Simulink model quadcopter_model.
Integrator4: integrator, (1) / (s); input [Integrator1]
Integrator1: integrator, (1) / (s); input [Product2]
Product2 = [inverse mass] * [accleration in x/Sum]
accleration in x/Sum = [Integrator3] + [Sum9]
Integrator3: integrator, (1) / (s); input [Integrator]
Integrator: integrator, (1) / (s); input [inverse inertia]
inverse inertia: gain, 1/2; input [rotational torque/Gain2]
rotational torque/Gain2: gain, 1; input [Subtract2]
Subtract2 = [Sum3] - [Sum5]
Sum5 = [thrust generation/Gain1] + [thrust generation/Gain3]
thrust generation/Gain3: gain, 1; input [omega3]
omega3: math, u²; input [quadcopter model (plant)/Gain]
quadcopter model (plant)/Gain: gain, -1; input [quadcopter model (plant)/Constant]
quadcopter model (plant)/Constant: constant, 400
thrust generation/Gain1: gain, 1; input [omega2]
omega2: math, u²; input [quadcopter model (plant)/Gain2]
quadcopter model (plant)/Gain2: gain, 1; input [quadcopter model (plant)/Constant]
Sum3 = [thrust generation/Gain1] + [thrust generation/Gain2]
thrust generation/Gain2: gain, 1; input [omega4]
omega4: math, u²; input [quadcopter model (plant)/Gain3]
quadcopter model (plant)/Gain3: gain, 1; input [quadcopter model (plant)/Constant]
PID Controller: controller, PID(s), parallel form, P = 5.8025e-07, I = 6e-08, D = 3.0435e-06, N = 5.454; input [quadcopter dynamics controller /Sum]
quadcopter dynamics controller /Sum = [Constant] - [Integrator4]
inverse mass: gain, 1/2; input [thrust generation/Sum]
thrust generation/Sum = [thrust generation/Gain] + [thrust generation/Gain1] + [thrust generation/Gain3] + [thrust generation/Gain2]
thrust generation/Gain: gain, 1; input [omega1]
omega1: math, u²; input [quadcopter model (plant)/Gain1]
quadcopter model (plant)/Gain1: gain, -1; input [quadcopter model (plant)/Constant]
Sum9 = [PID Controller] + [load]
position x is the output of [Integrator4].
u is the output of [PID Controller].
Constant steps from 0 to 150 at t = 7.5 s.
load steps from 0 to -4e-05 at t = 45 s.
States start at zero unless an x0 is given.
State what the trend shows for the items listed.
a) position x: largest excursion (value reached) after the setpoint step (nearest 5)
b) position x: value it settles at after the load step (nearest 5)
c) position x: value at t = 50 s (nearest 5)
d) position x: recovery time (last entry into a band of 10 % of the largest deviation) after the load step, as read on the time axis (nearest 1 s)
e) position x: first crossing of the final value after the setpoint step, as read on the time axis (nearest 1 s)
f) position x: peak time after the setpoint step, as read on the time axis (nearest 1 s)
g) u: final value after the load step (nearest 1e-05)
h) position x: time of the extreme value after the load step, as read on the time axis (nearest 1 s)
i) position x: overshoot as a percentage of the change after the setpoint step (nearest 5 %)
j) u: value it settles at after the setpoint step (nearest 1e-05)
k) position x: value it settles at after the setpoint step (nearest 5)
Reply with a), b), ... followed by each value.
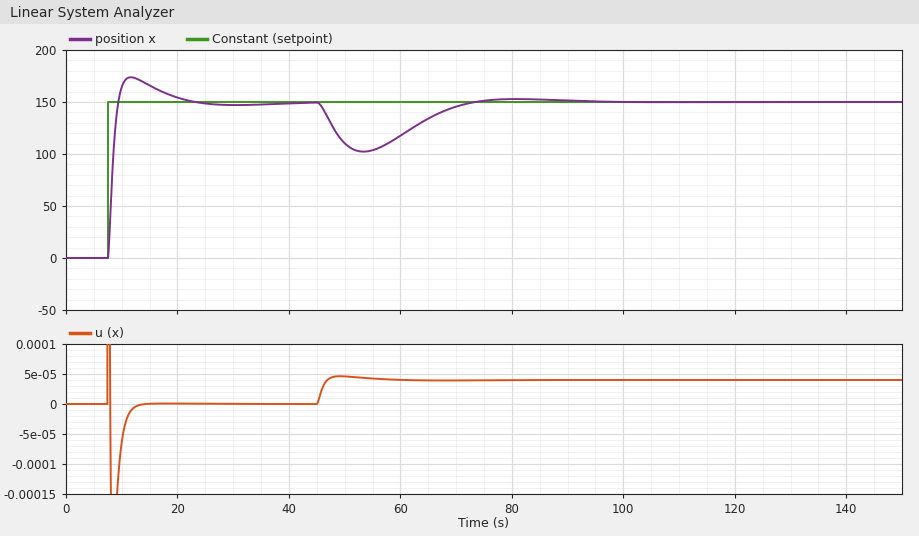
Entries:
a) 175
b) 150
c) 110
d) 70 s
e) 9 s
f) 12 s
g) 0.00004
h) 53 s
i) 15 %
j) 0.00000
k) 150
